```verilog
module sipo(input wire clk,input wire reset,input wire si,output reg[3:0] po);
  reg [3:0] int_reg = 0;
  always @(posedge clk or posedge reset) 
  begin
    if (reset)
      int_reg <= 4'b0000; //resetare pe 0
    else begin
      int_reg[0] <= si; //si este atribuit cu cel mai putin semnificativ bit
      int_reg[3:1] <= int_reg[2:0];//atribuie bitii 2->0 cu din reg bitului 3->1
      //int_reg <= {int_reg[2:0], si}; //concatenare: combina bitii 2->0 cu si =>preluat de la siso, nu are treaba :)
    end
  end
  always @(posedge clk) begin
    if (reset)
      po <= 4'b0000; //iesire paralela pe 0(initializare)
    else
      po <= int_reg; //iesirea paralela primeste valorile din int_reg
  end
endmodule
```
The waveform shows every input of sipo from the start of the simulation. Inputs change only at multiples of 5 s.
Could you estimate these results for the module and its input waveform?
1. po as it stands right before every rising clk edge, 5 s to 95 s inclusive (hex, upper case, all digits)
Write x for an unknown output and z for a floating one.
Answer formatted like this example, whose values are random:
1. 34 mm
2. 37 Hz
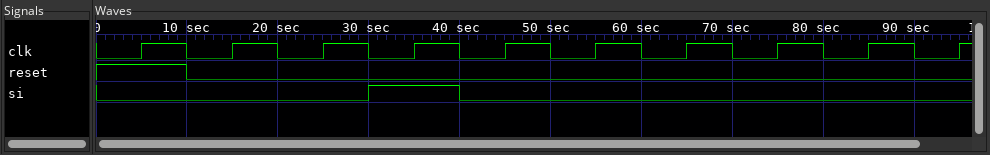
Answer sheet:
1. x, 0, 0, 0, 0, 1, 2, 4, 8, 0
